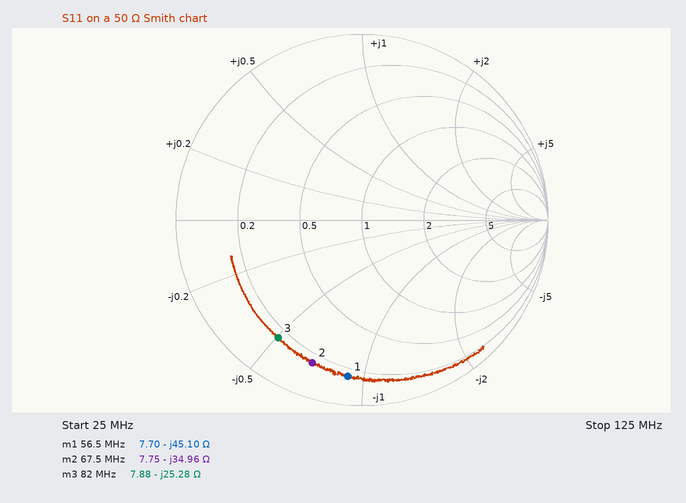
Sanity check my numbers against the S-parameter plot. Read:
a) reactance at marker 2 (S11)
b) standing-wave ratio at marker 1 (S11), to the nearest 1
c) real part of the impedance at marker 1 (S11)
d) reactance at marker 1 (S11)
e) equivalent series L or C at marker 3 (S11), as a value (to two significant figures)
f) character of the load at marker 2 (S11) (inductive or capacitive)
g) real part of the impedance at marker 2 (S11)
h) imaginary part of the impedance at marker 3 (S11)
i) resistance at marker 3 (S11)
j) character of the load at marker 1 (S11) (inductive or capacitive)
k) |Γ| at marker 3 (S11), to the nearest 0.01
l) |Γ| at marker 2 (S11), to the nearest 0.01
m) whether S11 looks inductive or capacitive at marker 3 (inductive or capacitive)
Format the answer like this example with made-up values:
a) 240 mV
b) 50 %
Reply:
a) -34.96 Ω
b) 12
c) 7.70 Ω
d) -45.10 Ω
e) 77 pF
f) capacitive
g) 7.75 Ω
h) -25.28 Ω
i) 7.88 Ω
j) capacitive
k) 0.78
l) 0.81
m) capacitive
